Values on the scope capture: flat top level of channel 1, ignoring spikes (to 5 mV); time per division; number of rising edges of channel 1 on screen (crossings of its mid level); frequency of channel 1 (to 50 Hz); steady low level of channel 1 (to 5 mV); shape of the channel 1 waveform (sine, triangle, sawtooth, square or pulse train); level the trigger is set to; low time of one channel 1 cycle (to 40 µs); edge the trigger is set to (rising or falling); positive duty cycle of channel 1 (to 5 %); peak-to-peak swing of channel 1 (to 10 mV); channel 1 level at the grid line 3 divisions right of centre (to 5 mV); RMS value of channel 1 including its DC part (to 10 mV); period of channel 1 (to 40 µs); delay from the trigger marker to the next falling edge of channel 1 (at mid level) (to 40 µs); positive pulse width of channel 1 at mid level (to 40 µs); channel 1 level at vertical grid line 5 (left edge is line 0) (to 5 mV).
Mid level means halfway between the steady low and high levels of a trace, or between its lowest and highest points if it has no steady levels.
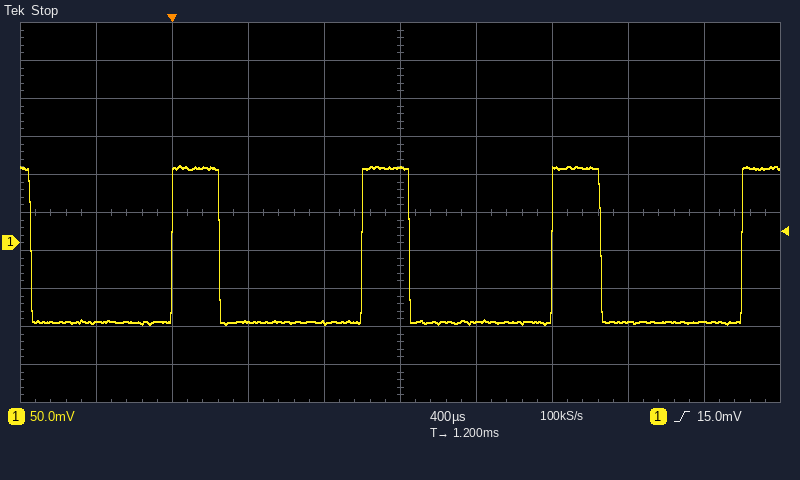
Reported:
100 mV
400 µs
4
1.00 kHz
-105 mV
pulse train
15.0 mV
760 µs
rising
25 %
210 mV
-105 mV
100 mV
1.00 ms
240 µs
240 µs
100 mV
